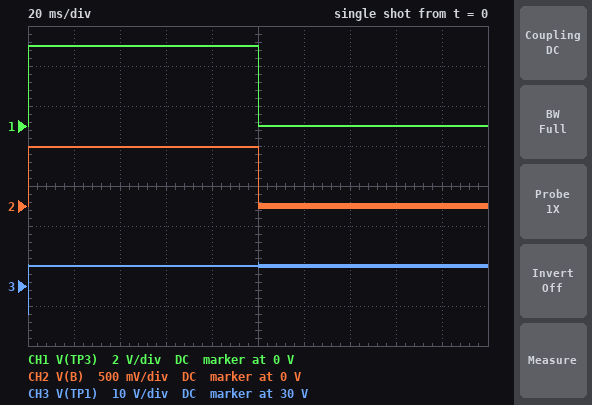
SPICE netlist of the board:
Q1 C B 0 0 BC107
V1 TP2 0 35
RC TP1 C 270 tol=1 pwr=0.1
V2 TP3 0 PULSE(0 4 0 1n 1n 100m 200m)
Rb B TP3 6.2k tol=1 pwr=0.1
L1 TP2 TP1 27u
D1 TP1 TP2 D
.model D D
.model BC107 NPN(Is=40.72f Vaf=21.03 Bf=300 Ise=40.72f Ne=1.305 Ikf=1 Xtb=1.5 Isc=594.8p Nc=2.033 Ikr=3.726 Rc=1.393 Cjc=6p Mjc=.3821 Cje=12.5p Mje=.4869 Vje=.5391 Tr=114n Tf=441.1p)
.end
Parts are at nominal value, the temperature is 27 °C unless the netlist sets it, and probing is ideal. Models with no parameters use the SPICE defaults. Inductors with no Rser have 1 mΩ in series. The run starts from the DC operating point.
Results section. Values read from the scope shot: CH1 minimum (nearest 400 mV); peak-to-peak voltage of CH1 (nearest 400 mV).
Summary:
0 V
4.0 V
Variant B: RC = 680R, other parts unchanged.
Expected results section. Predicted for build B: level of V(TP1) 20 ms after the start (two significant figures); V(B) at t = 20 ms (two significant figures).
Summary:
35 V
720 mV
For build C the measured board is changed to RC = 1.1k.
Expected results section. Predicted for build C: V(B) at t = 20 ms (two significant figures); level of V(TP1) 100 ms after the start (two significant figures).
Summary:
710 mV
35 V
